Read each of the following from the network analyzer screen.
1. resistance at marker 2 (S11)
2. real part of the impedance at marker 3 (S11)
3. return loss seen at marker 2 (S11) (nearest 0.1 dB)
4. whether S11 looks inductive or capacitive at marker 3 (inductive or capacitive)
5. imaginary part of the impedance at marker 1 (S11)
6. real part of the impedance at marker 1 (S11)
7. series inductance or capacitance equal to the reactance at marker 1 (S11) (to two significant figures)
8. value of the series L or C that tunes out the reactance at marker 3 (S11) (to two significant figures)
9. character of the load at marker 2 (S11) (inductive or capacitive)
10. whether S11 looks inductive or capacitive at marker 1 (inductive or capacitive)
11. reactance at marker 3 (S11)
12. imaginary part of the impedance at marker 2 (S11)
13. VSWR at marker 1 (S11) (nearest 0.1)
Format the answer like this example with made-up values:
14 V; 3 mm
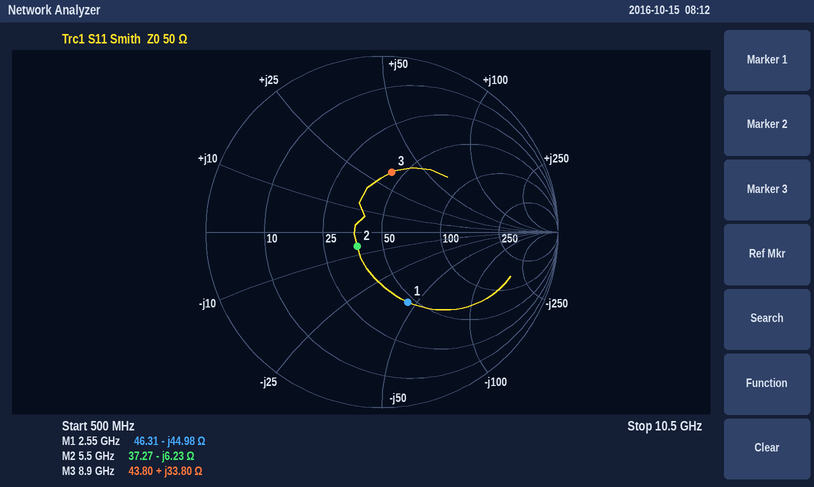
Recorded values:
37.27 Ω; 43.80 Ω; 15.8 dB; inductive; -44.98 Ω; 46.31 Ω; 1.4 pF; 530 fF; capacitive; capacitive; +33.80 Ω; -6.23 Ω; 2.5
